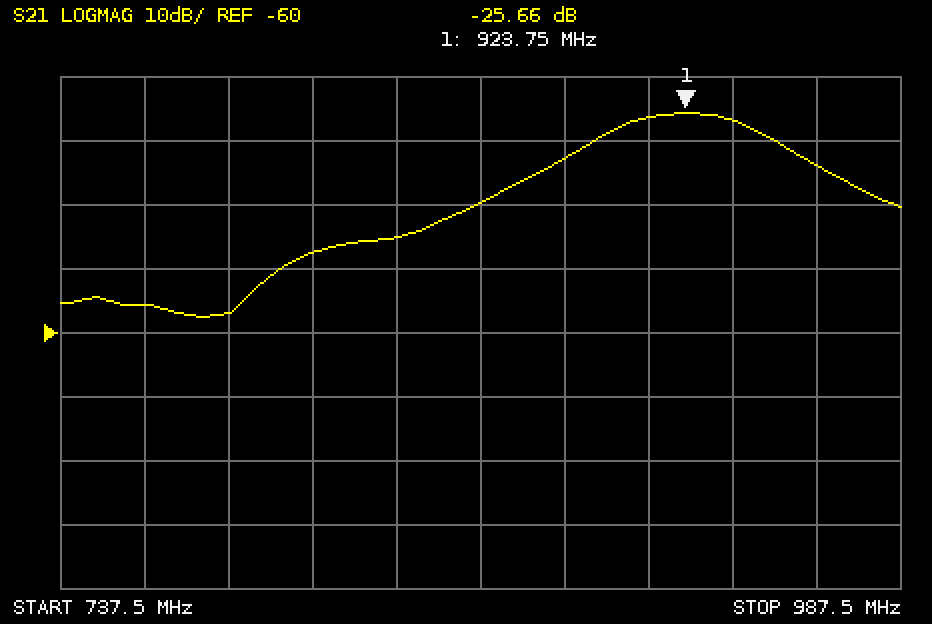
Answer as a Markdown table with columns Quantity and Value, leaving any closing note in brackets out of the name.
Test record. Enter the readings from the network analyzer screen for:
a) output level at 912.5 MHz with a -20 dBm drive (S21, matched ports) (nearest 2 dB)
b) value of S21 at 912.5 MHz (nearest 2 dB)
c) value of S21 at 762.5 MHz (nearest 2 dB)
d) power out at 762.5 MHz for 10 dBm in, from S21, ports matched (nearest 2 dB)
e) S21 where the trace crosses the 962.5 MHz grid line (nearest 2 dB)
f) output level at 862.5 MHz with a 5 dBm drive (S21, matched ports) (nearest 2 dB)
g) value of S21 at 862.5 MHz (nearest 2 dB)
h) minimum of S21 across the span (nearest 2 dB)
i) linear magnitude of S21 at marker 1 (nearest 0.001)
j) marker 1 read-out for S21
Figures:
| Quantity | Value |
|---|---|
| output level at 912.5 MHz with a -20 dBm drive (S21, matched ports) | -46 dBm |
| value of S21 at 912.5 MHz | -26 dB |
| value of S21 at 762.5 MHz | -56 dB |
| power out at 762.5 MHz for 10 dBm in, from S21, ports matched | -46 dBm |
| S21 where the trace crosses the 962.5 MHz grid line | -34 dB |
| output level at 862.5 MHz with a 5 dBm drive (S21, matched ports) | -34 dBm |
| value of S21 at 862.5 MHz | -40 dB |
| minimum of S21 across the span | -58 dB |
| linear magnitude of S21 at marker 1 | 0.052 |
| marker 1 read-out for S21 | -25.66 dB |
